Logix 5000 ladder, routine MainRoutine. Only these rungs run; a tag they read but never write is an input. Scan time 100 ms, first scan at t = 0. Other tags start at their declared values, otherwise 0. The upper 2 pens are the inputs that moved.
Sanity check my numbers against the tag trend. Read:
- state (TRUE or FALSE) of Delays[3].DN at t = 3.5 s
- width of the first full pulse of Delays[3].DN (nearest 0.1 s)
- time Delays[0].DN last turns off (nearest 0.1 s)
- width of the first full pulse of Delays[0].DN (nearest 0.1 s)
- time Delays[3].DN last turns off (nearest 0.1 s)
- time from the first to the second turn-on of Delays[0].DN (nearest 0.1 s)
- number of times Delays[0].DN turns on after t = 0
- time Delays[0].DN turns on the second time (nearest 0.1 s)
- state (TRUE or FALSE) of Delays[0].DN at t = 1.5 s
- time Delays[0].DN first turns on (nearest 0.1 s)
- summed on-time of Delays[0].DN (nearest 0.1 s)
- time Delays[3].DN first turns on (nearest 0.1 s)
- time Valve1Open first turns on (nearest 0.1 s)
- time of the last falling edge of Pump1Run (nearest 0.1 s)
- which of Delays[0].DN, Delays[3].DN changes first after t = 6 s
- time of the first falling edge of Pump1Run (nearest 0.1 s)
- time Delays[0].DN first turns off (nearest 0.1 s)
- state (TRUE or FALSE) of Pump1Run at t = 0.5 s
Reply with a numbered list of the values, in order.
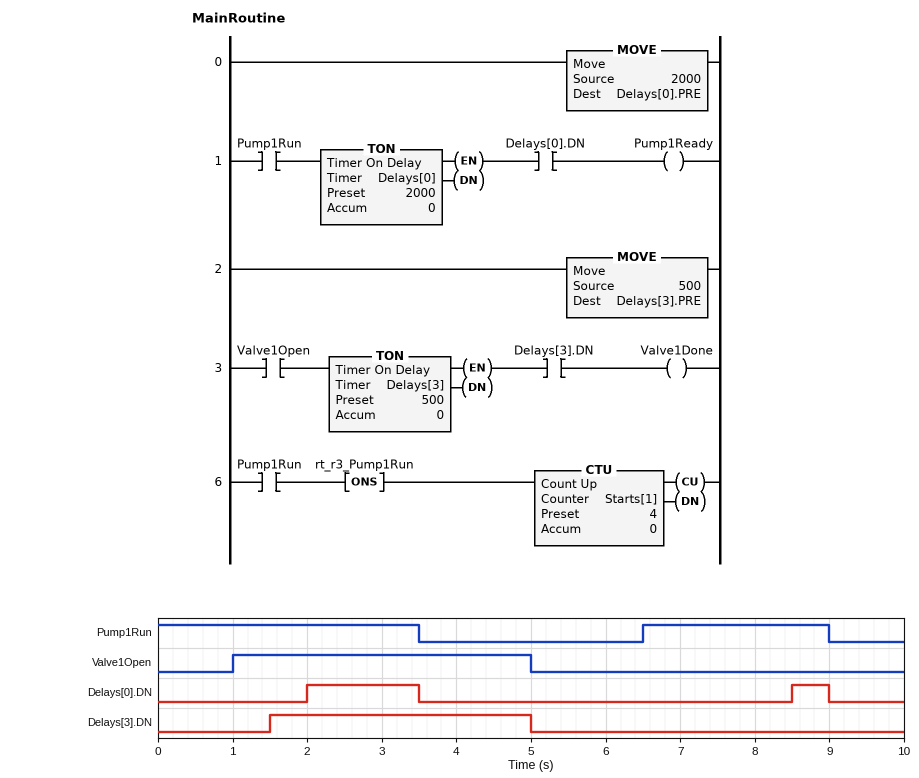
1. TRUE
2. 3.5 s
3. 9.0 s
4. 1.5 s
5. 5.0 s
6. 6.5 s
7. 2
8. 8.5 s
9. FALSE
10. 2.0 s
11. 2.0 s
12. 1.5 s
13. 1.0 s
14. 9.0 s
15. Delays[0].DN
16. 3.5 s
17. 3.5 s
18. TRUE
